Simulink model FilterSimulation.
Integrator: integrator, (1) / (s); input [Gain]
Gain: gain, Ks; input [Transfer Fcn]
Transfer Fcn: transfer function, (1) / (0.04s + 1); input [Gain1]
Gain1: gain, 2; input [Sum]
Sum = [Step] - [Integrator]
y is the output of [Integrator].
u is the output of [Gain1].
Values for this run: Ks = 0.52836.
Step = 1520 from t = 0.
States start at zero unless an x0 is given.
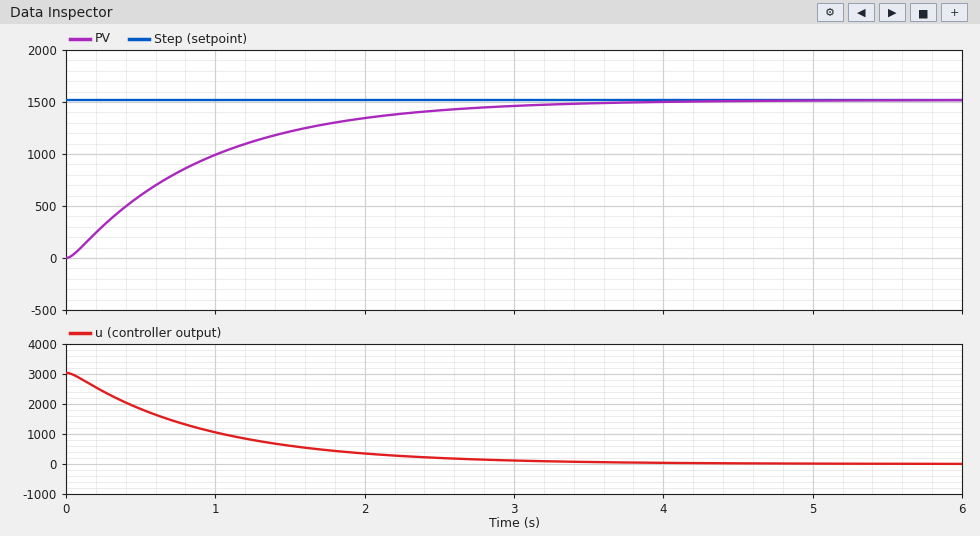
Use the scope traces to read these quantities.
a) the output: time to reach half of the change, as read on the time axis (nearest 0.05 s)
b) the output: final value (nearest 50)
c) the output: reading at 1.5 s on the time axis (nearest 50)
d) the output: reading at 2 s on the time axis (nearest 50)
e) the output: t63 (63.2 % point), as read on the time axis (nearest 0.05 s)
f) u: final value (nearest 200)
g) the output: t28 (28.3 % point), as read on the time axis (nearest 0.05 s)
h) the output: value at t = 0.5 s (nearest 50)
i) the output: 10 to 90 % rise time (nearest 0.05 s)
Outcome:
0.65 s
1500
1200
1350
0.95 s
0
0.35 s
600
2.00 s
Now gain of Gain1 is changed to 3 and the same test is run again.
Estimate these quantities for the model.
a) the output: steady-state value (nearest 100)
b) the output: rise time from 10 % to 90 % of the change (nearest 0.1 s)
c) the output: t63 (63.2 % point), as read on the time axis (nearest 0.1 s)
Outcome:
1500
1.3 s
0.6 s
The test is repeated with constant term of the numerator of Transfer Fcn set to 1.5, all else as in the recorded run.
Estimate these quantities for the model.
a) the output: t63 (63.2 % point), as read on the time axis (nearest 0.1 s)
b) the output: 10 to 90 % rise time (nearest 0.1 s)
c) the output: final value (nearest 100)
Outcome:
0.6 s
1.3 s
1500
